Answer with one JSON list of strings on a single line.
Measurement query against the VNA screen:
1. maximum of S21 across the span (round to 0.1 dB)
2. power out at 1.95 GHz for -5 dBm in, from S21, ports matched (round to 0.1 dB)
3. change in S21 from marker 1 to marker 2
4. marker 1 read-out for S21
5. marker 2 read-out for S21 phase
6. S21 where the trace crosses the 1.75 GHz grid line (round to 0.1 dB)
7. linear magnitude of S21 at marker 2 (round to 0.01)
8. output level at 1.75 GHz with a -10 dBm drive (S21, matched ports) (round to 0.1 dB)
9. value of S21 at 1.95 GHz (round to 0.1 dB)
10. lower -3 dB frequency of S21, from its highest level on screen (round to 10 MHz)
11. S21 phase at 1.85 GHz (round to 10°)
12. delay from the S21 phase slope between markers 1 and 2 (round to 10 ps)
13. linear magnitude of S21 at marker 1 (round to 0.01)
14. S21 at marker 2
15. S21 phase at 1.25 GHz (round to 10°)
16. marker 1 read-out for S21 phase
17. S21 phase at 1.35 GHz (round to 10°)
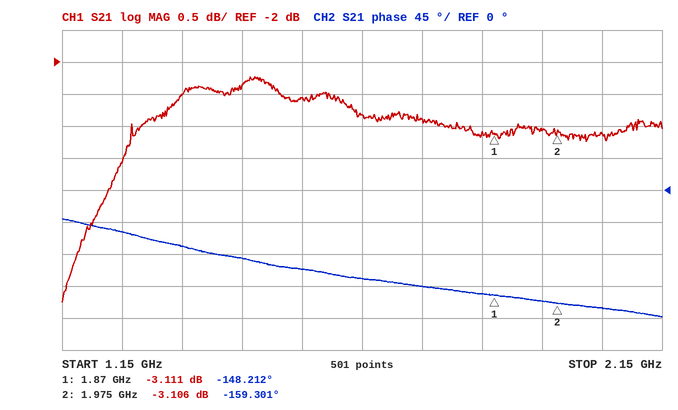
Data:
["-2.2 dB", "-8.1 dBm", "0.005 dB", "-3.111 dB", "-159.301°", "-2.9 dB", "0.70", "-12.9 dBm", "-3.1 dB", "1.17 GHz", "-150°", "290 ps", "0.70", "-3.106 dB", "-60°", "-148.212°", "-80°"]
